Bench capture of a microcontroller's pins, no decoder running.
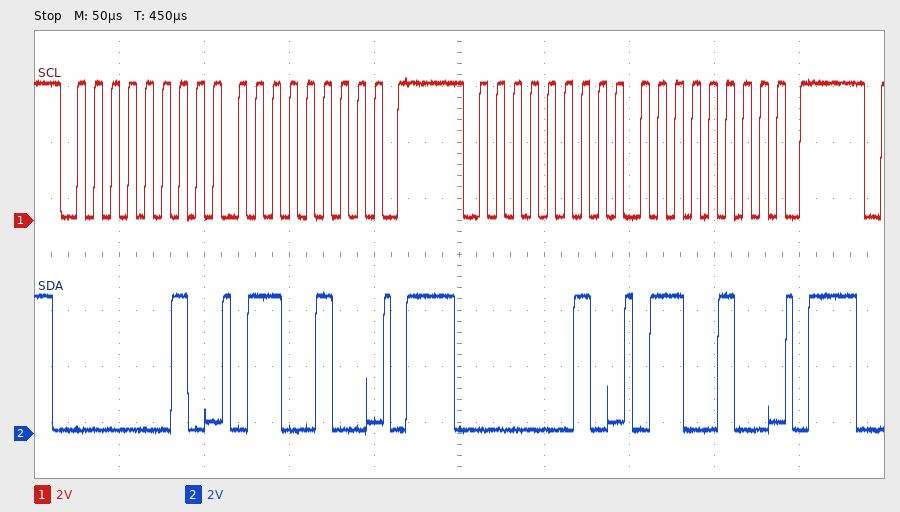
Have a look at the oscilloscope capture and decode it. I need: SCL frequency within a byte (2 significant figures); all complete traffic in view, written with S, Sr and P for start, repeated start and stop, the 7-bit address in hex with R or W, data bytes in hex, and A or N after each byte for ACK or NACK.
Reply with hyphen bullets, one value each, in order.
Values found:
- 100 kHz
- S 01W A 64 A P S 01W A 64 A P
